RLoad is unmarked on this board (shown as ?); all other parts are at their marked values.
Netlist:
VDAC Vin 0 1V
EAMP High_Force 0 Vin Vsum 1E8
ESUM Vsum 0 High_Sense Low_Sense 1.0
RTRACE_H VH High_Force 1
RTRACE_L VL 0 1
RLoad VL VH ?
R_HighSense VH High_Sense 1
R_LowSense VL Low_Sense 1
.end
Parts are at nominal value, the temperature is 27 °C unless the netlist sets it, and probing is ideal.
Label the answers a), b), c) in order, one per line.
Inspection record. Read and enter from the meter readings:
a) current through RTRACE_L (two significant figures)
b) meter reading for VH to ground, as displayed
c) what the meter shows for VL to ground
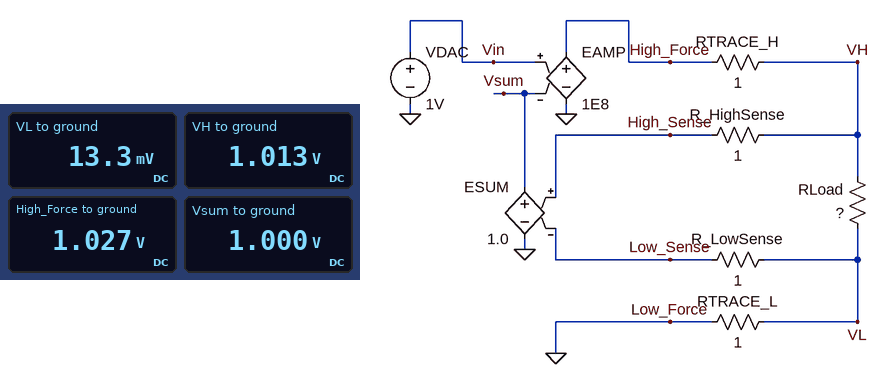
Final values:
a) 13 mA
b) 1.013 V
c) 13.3 mV
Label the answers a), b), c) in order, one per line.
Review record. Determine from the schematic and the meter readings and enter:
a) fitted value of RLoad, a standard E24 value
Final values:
a) 75 Ω
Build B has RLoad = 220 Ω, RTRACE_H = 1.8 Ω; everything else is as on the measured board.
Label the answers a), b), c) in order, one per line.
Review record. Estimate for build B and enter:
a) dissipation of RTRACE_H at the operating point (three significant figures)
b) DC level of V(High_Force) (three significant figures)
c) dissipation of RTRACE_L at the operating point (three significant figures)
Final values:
a) 37.2 µW
b) 1.01 V
c) 20.7 µW
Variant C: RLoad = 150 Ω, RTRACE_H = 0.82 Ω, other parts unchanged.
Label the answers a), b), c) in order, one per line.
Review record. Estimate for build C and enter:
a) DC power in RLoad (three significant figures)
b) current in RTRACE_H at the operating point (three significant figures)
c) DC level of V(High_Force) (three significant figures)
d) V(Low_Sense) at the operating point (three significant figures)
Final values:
a) 6.67 mW
b) 6.67 mA
c) 1.01 V
d) 6.67 mV
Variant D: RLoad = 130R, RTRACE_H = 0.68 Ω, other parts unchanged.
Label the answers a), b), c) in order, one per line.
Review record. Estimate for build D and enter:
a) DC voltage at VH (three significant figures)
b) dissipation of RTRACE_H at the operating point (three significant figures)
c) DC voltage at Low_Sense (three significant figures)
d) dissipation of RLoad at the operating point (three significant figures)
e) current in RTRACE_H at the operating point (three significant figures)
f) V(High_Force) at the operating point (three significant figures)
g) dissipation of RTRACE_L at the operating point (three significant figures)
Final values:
a) 1.01 V
b) 40.2 µW
c) 7.69 mV
d) 7.69 mW
e) 7.69 mA
f) 1.01 V
g) 59.2 µW
